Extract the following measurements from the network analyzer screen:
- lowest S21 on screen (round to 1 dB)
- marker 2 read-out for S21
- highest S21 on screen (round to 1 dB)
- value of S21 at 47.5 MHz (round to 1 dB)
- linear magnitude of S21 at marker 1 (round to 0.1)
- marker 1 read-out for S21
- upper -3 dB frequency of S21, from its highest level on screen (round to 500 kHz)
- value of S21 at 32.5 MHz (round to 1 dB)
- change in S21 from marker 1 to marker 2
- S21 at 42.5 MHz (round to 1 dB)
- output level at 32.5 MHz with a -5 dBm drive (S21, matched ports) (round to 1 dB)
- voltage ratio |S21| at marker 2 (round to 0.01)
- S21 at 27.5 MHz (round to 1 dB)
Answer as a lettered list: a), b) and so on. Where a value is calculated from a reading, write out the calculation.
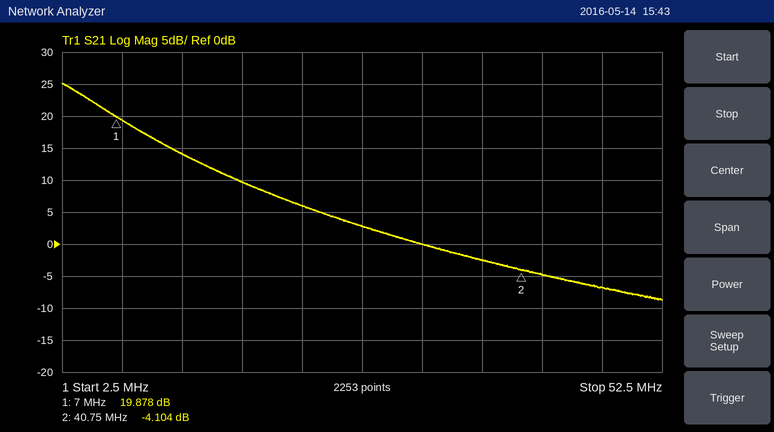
a) -9 dB
b) -4.104 dB
c) 25 dB
d) -7 dB
e) 10^(19.878/20) ≈ 9.9
f) 19.878 dB
g) 5.0 MHz
h) 0 dB
i) -4.104 − (19.878) = -23.982 dB
j) -5 dB
k) -5 dBm + (0 dB) = -5 dBm
l) 10^(-4.104/20) ≈ 0.62
m) 3 dB
